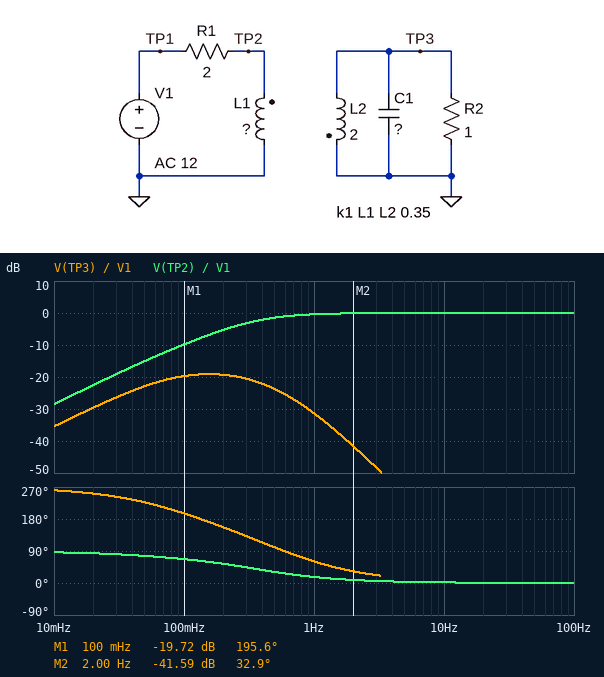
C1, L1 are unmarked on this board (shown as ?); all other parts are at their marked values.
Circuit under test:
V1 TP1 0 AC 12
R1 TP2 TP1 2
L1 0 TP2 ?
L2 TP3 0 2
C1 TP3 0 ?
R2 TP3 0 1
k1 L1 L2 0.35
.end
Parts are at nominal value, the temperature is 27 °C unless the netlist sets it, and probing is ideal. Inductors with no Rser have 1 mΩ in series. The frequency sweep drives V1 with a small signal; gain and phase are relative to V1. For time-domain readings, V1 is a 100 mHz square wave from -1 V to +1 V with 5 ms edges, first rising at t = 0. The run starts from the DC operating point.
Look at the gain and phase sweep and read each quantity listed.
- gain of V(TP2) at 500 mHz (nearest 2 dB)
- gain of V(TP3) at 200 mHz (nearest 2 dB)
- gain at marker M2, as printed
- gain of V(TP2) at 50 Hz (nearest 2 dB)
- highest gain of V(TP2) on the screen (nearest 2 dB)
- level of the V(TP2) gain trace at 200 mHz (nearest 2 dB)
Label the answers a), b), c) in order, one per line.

a) -2 dB
b) -20 dB
c) -41.59 dB
d) 0 dB
e) 0 dB
f) -6 dB
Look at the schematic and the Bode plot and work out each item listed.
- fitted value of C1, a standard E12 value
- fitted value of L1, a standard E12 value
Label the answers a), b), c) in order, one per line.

a) 180 mF
b) 1.2 H
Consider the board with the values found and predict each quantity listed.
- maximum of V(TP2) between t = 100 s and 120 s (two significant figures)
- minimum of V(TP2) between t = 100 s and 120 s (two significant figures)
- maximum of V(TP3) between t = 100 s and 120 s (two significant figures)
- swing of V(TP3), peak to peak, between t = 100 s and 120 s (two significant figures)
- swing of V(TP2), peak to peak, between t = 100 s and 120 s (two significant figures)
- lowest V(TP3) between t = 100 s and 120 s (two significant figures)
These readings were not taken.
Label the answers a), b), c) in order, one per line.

a) 2.0 V
b) -2.0 V
c) 160 mV
d) 310 mV
e) 4.0 V
f) -160 mV
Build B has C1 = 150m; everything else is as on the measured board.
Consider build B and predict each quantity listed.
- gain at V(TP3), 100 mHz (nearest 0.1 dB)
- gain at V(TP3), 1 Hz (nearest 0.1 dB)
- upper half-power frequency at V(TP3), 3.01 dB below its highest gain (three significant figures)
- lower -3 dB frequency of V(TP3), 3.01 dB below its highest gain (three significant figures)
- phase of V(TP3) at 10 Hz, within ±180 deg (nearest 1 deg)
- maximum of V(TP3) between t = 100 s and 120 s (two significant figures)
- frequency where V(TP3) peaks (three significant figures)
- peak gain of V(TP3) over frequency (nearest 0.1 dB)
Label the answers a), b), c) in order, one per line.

a) -19.8 dB
b) -30.5 dB
c) 414 mHz
d) 56.3 mHz
e) 8 deg
f) 160 mV
g) 157 mHz
h) -19.2 dB
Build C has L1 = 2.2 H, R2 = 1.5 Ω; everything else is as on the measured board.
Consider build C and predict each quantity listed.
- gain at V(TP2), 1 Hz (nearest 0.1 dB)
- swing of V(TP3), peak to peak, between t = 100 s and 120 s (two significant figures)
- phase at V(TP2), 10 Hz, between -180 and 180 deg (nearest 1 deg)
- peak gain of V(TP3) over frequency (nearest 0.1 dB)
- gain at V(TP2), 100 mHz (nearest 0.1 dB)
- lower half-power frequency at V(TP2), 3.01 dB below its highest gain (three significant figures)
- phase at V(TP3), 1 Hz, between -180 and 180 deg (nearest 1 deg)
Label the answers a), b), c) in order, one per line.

a) -0.1 dB
b) 470 mV
c) 1 deg
d) -15.5 dB
e) -5.5 dB
f) 172 mHz
g) 42 deg
